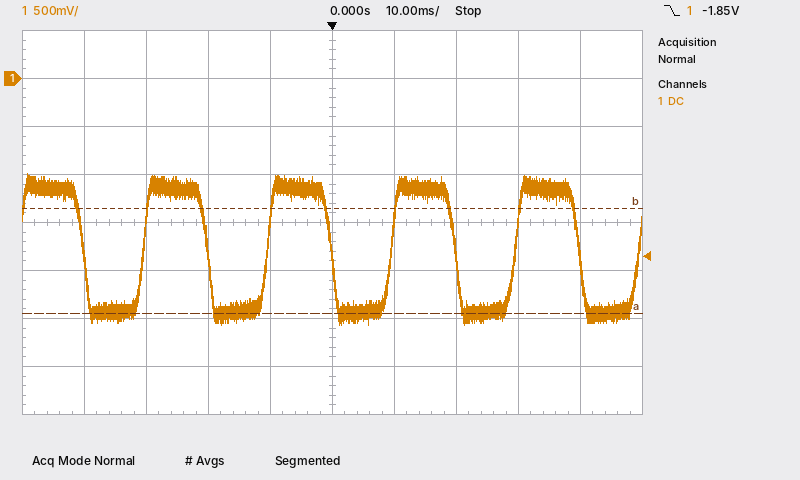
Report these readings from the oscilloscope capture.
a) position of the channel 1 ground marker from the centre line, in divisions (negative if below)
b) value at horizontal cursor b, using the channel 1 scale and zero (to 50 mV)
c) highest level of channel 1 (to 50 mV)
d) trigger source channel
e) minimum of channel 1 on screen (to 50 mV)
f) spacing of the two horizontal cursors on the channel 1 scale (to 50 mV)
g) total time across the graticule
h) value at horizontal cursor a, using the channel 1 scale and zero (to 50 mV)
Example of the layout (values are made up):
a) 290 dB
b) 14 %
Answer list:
a) +3.0 div
b) -1.35 V
c) -1.00 V
d) channel 1
e) -2.55 V
f) 1.10 V
g) 100 ms
h) -2.45 V
